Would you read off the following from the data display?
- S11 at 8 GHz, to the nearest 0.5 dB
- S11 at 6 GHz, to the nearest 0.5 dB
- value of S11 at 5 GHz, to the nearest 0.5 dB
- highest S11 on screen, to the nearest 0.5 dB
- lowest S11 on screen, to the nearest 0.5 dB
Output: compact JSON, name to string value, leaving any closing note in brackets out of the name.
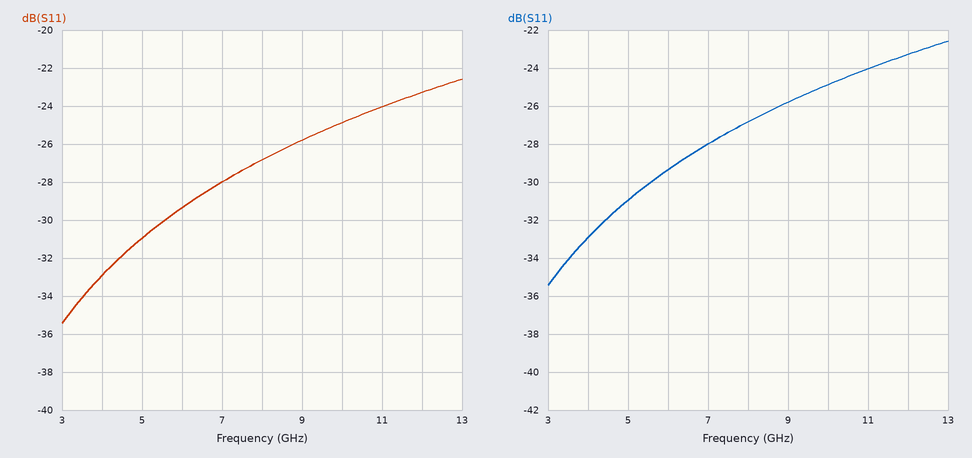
{"S11 at 8 GHz, to the nearest 0.5 dB": "-27.0 dB", "S11 at 6 GHz, to the nearest 0.5 dB": "-29.5 dB", "value of S11 at 5 GHz, to the nearest 0.5 dB": "-31.0 dB", "highest S11 on screen, to the nearest 0.5 dB": "-22.5 dB", "lowest S11 on screen, to the nearest 0.5 dB": "-35.5 dB"}
